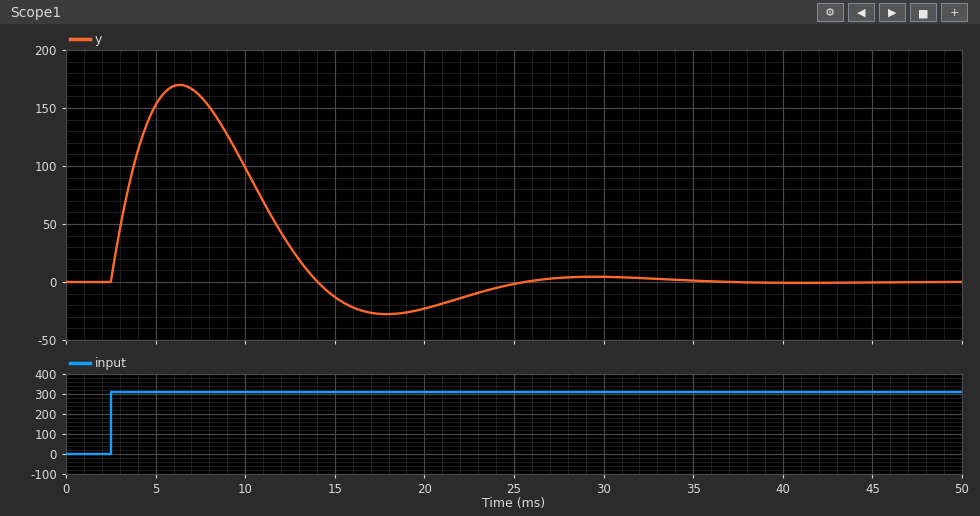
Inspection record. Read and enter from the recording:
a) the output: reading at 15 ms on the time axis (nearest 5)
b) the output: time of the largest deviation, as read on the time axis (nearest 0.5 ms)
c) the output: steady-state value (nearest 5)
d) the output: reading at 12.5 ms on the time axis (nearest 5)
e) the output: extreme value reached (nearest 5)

-15
6.5 ms
0
30
170
